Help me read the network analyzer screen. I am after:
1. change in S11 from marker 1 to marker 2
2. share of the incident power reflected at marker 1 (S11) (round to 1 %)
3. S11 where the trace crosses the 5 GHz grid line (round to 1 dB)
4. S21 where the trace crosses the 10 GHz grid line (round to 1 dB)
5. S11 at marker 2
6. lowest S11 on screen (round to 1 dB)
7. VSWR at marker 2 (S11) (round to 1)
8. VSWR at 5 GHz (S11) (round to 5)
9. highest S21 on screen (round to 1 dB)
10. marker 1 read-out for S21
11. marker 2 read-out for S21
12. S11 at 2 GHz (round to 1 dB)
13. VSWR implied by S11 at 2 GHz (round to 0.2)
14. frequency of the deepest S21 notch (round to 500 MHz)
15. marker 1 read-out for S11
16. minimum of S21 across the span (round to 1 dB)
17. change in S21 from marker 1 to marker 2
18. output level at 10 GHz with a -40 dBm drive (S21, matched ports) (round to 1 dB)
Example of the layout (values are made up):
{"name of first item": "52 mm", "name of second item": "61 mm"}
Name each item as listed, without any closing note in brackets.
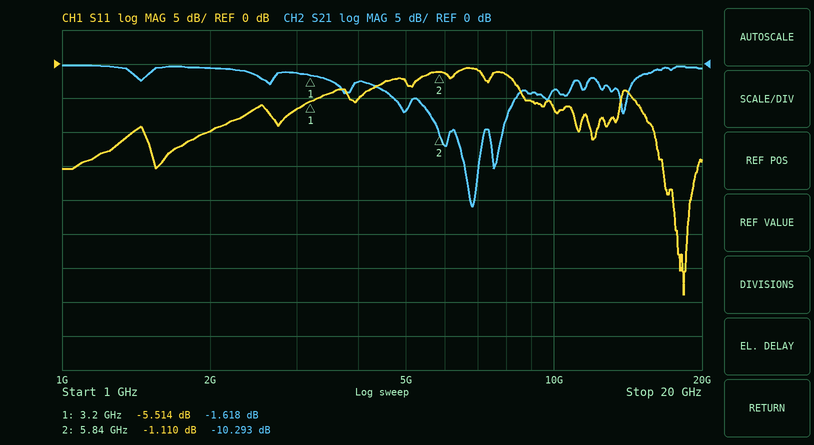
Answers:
{"change in S11 from marker 1 to marker 2": "4.404 dB", "share of the incident power reflected at marker 1 (S11)": "28 %", "S11 where the trace crosses the 5 GHz grid line": "-3 dB", "S21 where the trace crosses the 10 GHz grid line": "-4 dB", "S11 at marker 2": "-1.110 dB", "lowest S11 on screen": "-34 dB", "VSWR at marker 2 (S11)": "16", "VSWR at 5 GHz (S11)": "5", "highest S21 on screen": "0 dB", "marker 1 read-out for S21": "-1.618 dB", "marker 2 read-out for S21": "-10.293 dB", "S11 at 2 GHz": "-10 dB", "VSWR implied by S11 at 2 GHz": "2.0", "frequency of the deepest S21 notch": "7.0 GHz", "marker 1 read-out for S11": "-5.514 dB", "minimum of S21 across the span": "-21 dB", "change in S21 from marker 1 to marker 2": "-8.675 dB", "output level at 10 GHz with a -40 dBm drive (S21, matched ports)": "-44 dBm"}
